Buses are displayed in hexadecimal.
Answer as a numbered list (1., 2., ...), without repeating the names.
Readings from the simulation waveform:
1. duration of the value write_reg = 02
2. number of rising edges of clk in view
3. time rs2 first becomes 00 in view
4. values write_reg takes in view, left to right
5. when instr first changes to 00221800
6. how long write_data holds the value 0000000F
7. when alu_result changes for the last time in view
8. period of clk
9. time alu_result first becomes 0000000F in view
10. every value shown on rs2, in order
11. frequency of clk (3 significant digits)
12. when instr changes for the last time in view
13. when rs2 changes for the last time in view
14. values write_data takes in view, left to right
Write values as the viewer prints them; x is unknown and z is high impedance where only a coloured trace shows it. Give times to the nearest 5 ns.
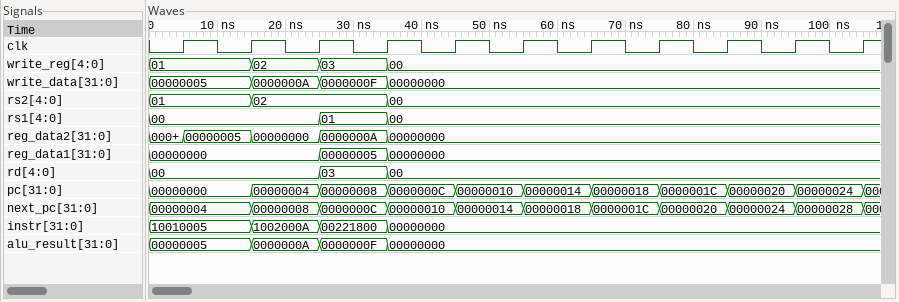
1. 10 ns
2. 11
3. 35 ns
4. 01, 02, 03, 00
5. 25 ns
6. 10 ns
7. 35 ns
8. 10 ns
9. 25 ns
10. 01, 02, 00
11. 100 MHz
12. 35 ns
13. 35 ns
14. 00000005, 0000000A, 0000000F, 00000000
